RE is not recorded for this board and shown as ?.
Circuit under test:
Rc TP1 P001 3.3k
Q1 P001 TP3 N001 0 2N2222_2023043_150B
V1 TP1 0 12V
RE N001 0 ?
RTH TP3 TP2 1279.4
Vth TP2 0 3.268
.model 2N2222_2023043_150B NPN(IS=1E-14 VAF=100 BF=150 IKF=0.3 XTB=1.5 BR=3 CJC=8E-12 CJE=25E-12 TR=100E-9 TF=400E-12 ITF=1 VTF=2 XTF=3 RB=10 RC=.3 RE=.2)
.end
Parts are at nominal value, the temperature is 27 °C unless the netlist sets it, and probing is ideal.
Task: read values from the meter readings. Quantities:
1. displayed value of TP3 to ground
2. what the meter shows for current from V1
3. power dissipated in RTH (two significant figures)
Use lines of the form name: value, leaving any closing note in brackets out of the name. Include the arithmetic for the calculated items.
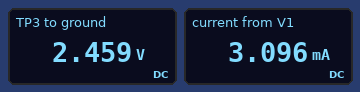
displayed value of TP3 to ground: 2.459 V
what the meter shows for current from V1: 3.096 mA
power dissipated in RTH: (3.268 V - 2.459 V)^2 / 1.279 kΩ = 510 µW
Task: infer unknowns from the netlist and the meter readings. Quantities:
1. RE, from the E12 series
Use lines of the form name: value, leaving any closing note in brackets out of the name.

RE, from the E12 series: 470 Ω
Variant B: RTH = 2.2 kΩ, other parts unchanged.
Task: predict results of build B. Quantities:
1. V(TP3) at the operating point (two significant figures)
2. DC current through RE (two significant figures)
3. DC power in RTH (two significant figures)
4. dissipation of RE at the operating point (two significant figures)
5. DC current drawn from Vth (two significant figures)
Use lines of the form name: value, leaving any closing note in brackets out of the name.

V(TP3) at the operating point: 2.4 V
DC current through RE: 3.5 mA
DC power in RTH: 370 µW
dissipation of RE at the operating point: 5.9 mW
DC current drawn from Vth: 410 µA
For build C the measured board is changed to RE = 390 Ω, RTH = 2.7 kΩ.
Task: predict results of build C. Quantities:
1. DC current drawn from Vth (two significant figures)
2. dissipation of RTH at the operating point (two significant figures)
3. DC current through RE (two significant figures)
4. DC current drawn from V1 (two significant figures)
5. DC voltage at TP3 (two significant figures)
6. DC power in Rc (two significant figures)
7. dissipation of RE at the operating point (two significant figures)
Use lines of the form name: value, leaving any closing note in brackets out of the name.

DC current drawn from Vth: 430 µA
dissipation of RTH at the operating point: 490 µW
DC current through RE: 3.6 mA
DC current drawn from V1: 3.2 mA
DC voltage at TP3: 2.1 V
DC power in Rc: 34 mW
dissipation of RE at the operating point: 5.1 mW
